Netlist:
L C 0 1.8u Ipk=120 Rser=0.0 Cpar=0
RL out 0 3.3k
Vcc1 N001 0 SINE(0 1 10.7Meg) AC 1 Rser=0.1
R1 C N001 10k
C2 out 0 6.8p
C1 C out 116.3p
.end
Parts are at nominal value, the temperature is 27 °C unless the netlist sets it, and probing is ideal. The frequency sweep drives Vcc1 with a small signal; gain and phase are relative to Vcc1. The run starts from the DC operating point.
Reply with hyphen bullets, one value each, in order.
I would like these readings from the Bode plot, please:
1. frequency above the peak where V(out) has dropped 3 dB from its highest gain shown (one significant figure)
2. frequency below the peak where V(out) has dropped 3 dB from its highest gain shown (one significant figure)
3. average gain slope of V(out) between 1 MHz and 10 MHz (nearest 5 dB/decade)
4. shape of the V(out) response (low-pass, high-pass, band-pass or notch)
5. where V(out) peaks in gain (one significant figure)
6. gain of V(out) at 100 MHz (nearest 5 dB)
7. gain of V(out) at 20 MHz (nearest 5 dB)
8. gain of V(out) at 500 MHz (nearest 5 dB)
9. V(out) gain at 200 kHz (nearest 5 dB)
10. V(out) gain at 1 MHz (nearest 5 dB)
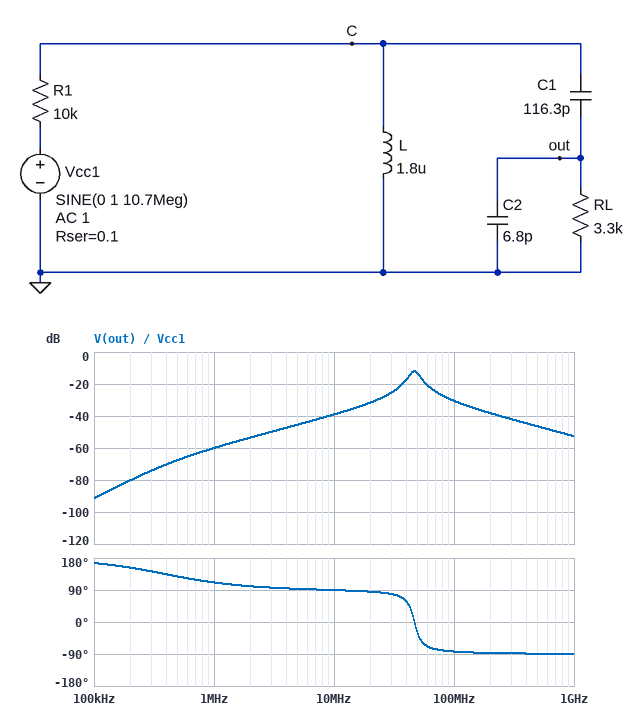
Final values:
- 50 MHz
- 40 MHz
- 20 dB/decade
- band-pass
- 50 MHz
- -30 dB
- -30 dB
- -45 dB
- -80 dB
- -60 dB
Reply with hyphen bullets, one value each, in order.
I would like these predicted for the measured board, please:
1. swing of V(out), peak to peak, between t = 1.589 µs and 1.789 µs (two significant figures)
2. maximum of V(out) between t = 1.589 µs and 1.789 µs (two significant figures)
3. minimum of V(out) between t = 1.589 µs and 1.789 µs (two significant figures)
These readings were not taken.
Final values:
- 24 mV
- 12 mV
- -12 mV
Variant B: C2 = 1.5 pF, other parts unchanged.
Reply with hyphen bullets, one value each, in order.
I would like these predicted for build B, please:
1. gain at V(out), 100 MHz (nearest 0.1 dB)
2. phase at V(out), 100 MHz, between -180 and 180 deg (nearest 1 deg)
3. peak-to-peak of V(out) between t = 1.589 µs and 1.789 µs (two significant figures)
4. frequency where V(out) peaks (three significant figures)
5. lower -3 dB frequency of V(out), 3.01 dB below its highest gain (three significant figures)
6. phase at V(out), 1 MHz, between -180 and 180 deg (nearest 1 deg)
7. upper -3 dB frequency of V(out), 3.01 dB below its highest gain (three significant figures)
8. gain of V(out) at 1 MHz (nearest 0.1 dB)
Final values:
- -12.1 dB
- -7 deg
- 24 mV
- 97.4 MHz
- 78.5 MHz
- 112 deg
- 121 MHz
- -59.7 dB
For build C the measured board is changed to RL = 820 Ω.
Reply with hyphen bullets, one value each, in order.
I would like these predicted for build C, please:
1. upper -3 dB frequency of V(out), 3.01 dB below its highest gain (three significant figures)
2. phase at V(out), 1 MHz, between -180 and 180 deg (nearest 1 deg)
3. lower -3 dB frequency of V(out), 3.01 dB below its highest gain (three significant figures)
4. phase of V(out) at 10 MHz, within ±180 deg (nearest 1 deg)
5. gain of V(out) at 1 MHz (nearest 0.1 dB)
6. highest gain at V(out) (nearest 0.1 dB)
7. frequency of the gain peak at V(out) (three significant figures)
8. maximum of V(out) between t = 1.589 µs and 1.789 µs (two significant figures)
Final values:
- 63.3 MHz
- 147 deg
- 33.9 MHz
- 91 deg
- -64.8 dB
- -22.0 dB
- 46.3 MHz
- 12 mV
